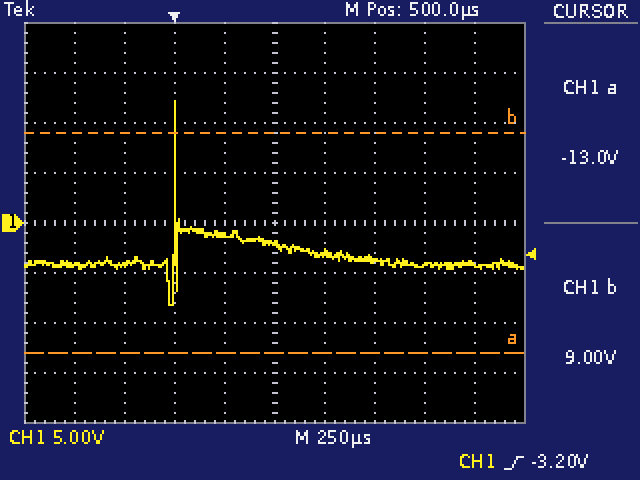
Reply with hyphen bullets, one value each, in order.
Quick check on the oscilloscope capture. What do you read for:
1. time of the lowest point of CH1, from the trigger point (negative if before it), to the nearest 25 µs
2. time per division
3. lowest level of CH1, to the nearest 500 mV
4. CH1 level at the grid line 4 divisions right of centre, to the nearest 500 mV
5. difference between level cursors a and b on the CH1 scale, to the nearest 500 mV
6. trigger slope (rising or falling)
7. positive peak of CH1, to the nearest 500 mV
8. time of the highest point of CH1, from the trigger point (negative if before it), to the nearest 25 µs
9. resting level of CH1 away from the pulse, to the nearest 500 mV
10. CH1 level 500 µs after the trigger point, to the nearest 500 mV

- -25 µs
- 250 µs
- -8.0 V
- -4.0 V
- 22.0 V
- rising
- 12.0 V
- 0 µs
- -4.0 V
- -2.0 V
